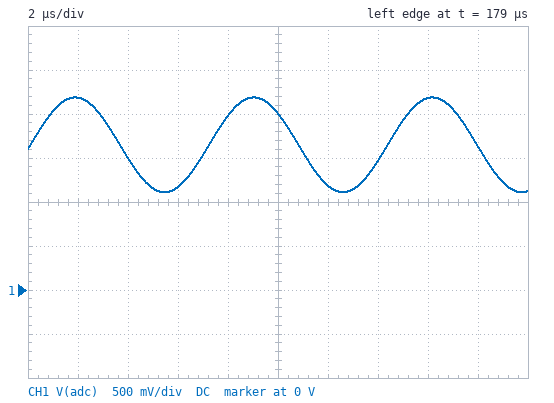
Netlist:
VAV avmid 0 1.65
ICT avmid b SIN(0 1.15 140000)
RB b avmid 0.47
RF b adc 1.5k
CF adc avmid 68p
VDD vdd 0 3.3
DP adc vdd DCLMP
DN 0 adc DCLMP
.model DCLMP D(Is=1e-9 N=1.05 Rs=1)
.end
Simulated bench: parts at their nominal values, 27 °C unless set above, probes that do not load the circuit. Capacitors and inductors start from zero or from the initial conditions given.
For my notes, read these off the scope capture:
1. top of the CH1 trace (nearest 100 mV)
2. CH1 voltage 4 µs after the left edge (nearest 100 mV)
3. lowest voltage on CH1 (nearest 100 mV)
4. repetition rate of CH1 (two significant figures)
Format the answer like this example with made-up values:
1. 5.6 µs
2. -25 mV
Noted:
1. 2.2 V
2. 1.5 V
3. 1.1 V
4. 140 kHz
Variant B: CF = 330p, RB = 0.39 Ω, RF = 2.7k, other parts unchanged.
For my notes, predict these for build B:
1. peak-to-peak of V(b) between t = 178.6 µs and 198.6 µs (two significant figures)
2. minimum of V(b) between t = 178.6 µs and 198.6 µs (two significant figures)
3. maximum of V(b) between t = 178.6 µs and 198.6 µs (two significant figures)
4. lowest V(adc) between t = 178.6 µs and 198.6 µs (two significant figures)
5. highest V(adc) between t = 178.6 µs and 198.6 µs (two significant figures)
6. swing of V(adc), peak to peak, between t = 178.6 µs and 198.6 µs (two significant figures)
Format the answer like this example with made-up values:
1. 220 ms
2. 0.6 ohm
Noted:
1. 900 mV
2. 1.2 V
3. 2.1 V
4. 1.3 V
5. 2.0 V
6. 710 mV
